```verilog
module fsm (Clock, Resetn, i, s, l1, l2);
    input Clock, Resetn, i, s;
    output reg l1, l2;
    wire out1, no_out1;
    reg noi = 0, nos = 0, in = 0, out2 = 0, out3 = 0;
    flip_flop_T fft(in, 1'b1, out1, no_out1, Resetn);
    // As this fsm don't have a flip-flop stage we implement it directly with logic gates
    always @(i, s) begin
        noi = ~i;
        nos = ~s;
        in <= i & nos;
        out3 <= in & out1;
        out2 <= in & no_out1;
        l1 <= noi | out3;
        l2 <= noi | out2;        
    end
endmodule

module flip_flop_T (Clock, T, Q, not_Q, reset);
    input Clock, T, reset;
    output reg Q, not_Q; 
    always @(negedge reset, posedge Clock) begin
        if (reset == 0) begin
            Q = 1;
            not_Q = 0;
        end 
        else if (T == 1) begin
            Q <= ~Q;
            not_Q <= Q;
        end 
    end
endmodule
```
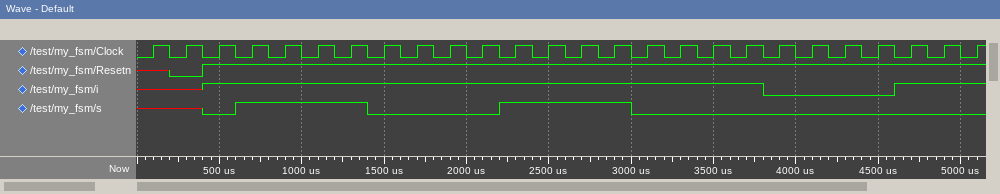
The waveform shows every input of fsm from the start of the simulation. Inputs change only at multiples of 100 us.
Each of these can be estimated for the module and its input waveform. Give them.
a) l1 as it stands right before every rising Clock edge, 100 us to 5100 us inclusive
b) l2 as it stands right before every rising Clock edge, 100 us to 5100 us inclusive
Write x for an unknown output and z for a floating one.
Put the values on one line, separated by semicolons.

x x 0 0 0 0 0 0 0 0 0 0 0 0 0 1 1 1 1 1 1 1 1 0 0 0; x x 0 0 0 0 0 1 1 1 1 0 0 0 0 0 0 0 0 1 1 1 1 1 1 1
